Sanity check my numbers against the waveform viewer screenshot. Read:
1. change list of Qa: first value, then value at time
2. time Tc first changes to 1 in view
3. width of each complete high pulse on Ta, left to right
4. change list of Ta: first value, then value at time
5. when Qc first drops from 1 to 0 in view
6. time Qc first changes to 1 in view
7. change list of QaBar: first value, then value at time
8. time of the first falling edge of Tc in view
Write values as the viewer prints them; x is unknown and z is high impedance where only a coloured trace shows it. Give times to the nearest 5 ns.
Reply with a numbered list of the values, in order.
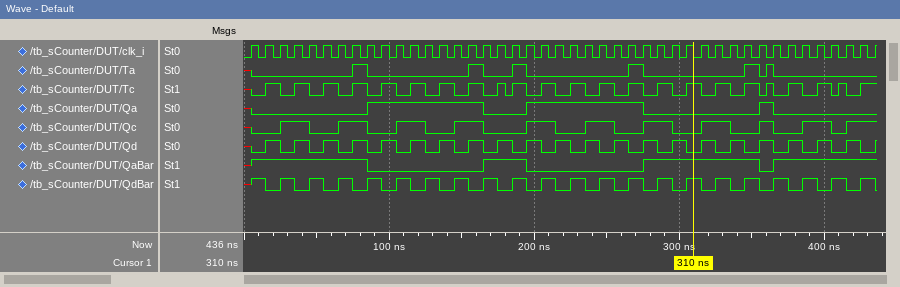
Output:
1. x, 0 at 5 ns, 1 at 85 ns, 0 at 165 ns, 1 at 195 ns, 0 at 275 ns, 1 at 355 ns, 0 at 365 ns
2. 15 ns
3. 10 ns, 10 ns, 10 ns, 10 ns, 10 ns, 5 ns
4. x, 0 at 5 ns, 1 at 75 ns, 0 at 85 ns, 1 at 155 ns, 0 at 165 ns, 1 at 185 ns, 0 at 195 ns, 1 at 265 ns, 0 at 275 ns, 1 at 345 ns, 0 at 355 ns, 1 at 360 ns, 0 at 365 ns
5. 45 ns
6. 25 ns
7. x, 1 at 5 ns, 0 at 85 ns, 1 at 165 ns, 0 at 195 ns, 1 at 275 ns, 0 at 355 ns, 1 at 365 ns
8. 25 ns
